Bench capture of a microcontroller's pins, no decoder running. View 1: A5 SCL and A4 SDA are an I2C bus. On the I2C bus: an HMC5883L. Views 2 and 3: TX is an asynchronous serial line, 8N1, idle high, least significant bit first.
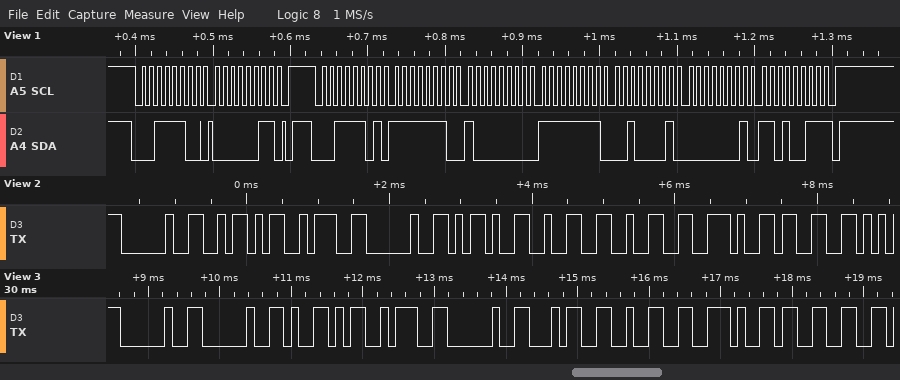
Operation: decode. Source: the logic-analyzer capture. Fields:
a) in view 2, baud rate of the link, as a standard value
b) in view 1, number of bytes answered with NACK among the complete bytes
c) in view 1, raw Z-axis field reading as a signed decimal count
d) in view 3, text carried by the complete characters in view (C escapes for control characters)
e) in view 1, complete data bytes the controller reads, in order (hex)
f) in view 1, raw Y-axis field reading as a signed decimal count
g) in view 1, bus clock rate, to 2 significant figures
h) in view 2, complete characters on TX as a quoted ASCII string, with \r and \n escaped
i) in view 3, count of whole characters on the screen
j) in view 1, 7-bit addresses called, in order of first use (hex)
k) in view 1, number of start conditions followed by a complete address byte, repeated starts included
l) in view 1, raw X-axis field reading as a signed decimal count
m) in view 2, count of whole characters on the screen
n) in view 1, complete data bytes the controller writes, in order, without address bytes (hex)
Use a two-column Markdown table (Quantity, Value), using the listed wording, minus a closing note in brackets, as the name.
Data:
| Quantity | Value |
|---|---|
| in view 2, baud rate of the link, as a standard value | 9600 baud |
| in view 1, number of bytes answered with NACK among the complete bytes | 1 |
| in view 1, raw Z-axis field reading as a signed decimal count | -223 |
| in view 3, text carried by the complete characters in view | "  Y: 42.3" |
| in view 1, complete data bytes the controller reads, in order | FE 80 FF 21 01 D3 |
| in view 1, raw Y-axis field reading as a signed decimal count | 467 |
| in view 1, bus clock rate, to 2 significant figures | 100 kHz |
| in view 2, complete characters on TX as a quoted ASCII string, with \r and \n escaped | " Z: -22.3" |
| in view 3, count of whole characters on the screen | 9 |
| in view 1, 7-bit addresses called, in order of first use | 0x1E |
| in view 1, number of start conditions followed by a complete address byte, repeated starts included | 2 |
| in view 1, raw X-axis field reading as a signed decimal count | -384 |
| in view 2, count of whole characters on the screen | 9 |
| in view 1, complete data bytes the controller writes, in order, without address bytes | 03 |
